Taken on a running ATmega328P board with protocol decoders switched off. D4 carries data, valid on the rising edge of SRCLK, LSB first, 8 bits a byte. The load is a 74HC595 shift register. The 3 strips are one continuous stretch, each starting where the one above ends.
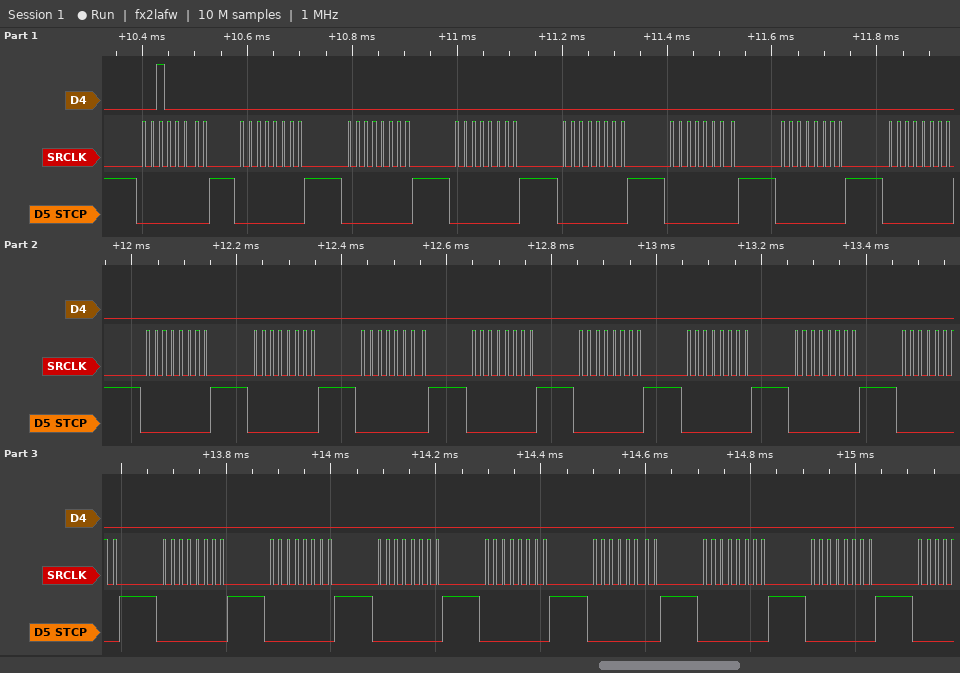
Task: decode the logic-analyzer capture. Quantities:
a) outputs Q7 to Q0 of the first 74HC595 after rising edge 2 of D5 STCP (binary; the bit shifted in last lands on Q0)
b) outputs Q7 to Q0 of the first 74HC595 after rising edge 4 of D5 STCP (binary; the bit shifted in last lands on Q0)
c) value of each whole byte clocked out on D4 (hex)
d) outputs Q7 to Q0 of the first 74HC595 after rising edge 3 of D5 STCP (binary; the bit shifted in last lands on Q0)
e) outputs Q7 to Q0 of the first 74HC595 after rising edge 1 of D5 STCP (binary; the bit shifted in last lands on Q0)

00000000
00000000
04 00 00 00 00 00 00 00 00 00 00 00 00 00 00 00 00 00 00 00 00 00 00
00000000
00100000
